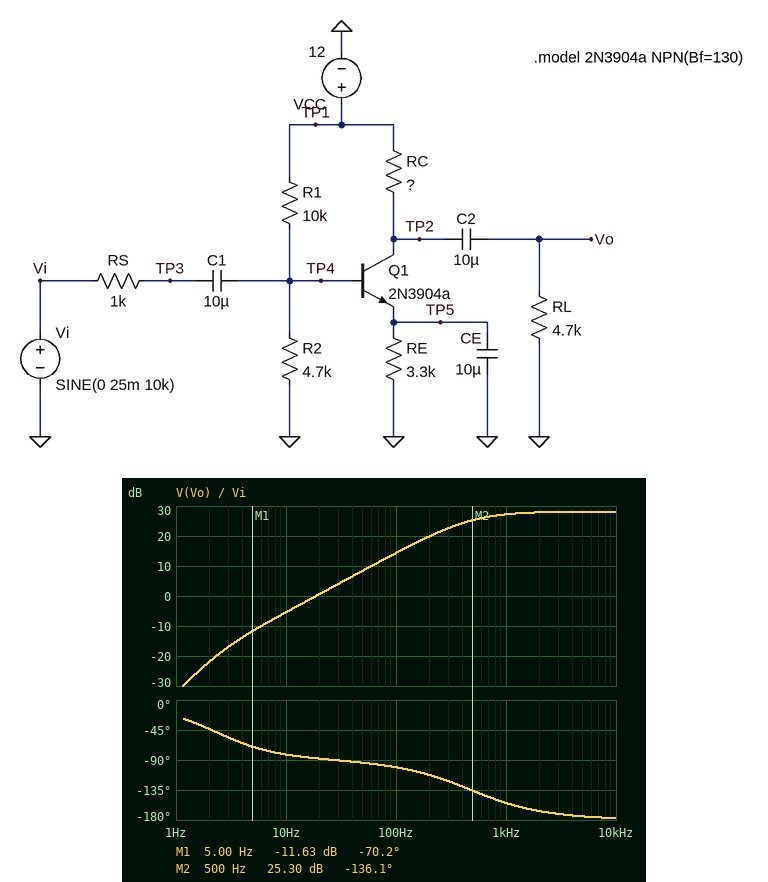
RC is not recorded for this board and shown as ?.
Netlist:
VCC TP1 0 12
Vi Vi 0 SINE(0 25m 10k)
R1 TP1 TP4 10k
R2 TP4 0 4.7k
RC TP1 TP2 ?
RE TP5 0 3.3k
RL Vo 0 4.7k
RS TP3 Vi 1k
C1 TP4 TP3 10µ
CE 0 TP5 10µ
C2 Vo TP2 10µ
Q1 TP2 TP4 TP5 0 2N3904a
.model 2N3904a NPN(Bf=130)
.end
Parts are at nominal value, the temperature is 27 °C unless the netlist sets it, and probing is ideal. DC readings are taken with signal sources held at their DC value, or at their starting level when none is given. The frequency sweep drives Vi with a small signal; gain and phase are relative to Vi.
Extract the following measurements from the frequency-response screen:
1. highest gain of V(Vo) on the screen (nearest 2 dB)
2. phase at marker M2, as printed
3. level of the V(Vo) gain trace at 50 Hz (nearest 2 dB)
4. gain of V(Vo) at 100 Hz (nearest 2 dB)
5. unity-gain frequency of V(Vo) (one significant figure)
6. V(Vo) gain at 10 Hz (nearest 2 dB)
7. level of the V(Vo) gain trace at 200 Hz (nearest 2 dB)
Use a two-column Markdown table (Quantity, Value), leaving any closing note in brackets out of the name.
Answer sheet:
| Quantity | Value |
|---|---|
| highest gain of V(Vo) on the screen | 28 dB |
| phase at marker M2, as printed | -136.1 deg |
| level of the V(Vo) gain trace at 50 Hz | 8 dB |
| gain of V(Vo) at 100 Hz | 14 dB |
| unity-gain frequency of V(Vo) | 20 Hz |
| V(Vo) gain at 10 Hz | -6 dB |
| level of the V(Vo) gain trace at 200 Hz | 20 dB |
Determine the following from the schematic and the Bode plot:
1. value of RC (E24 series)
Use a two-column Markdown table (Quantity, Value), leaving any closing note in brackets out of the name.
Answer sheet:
| Quantity | Value |
|---|---|
| value of RC | 1.5 kΩ |
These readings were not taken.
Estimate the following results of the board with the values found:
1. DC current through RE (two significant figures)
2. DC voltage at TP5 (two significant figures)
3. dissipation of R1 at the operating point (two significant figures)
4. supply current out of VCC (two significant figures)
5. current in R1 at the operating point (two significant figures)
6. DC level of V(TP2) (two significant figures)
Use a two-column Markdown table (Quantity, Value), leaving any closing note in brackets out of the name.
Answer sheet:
| Quantity | Value |
|---|---|
| DC current through RE | 920 µA |
| DC voltage at TP5 | 3.0 V |
| dissipation of R1 at the operating point | 6.7 mW |
| supply current out of VCC | 1.7 mA |
| current in R1 at the operating point | 820 µA |
| DC level of V(TP2) | 11 V |
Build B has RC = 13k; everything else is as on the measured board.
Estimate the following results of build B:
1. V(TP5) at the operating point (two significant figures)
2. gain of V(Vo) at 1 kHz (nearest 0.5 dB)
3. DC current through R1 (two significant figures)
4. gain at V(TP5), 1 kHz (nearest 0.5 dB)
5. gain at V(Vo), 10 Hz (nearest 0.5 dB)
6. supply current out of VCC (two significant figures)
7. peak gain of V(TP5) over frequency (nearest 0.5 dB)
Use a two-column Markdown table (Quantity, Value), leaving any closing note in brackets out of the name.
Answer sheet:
| Quantity | Value |
|---|---|
| V(TP5) at the operating point | 2.7 V |
| gain of V(Vo) at 1 kHz | -15.0 dB |
| DC current through R1 | 850 µA |
| gain at V(TP5), 1 kHz | -36.0 dB |
| gain at V(Vo), 10 Hz | -11.0 dB |
| supply current out of VCC | 1.6 mA |
| peak gain of V(TP5) over frequency | -9.5 dB |
